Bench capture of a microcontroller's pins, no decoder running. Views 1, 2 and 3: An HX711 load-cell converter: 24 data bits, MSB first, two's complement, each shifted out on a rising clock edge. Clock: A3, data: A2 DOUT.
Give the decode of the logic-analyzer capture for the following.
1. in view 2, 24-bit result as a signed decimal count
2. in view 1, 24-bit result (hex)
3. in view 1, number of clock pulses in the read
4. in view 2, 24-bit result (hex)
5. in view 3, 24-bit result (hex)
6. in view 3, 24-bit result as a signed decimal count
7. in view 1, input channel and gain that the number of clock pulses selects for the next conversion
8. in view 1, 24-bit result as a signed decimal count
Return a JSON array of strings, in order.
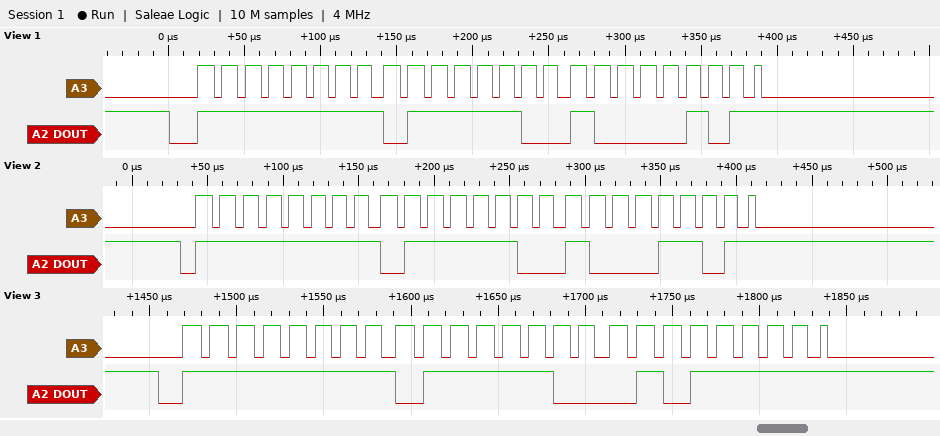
["-33651", "0xFF7C85", "25", "0xFF7C8D", "0xFF7C5F", "-33697", "channel A, gain 128", "-33659"]
